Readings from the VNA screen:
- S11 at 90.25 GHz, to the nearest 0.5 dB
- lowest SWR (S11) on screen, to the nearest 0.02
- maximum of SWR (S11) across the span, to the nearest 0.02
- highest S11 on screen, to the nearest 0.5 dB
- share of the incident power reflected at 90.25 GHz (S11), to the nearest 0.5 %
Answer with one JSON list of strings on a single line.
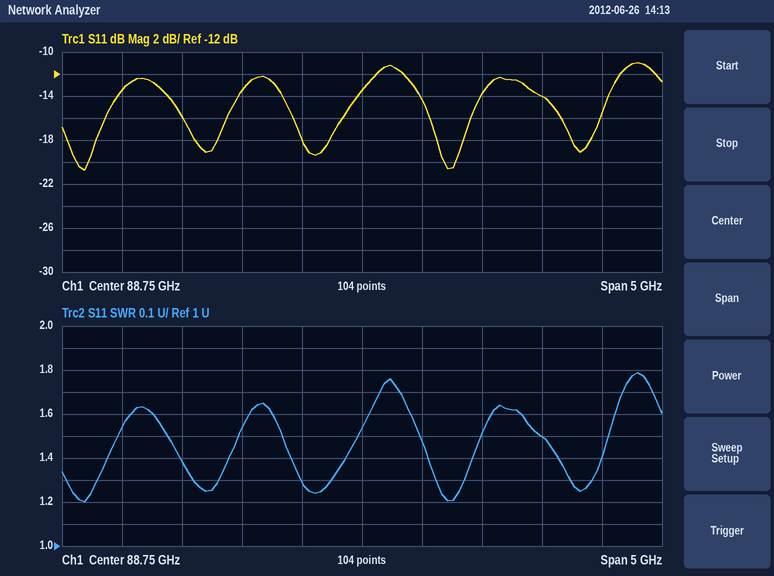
["-14.0 dB", "1.20", "1.78", "-11.0 dB", "4.0 %"]
